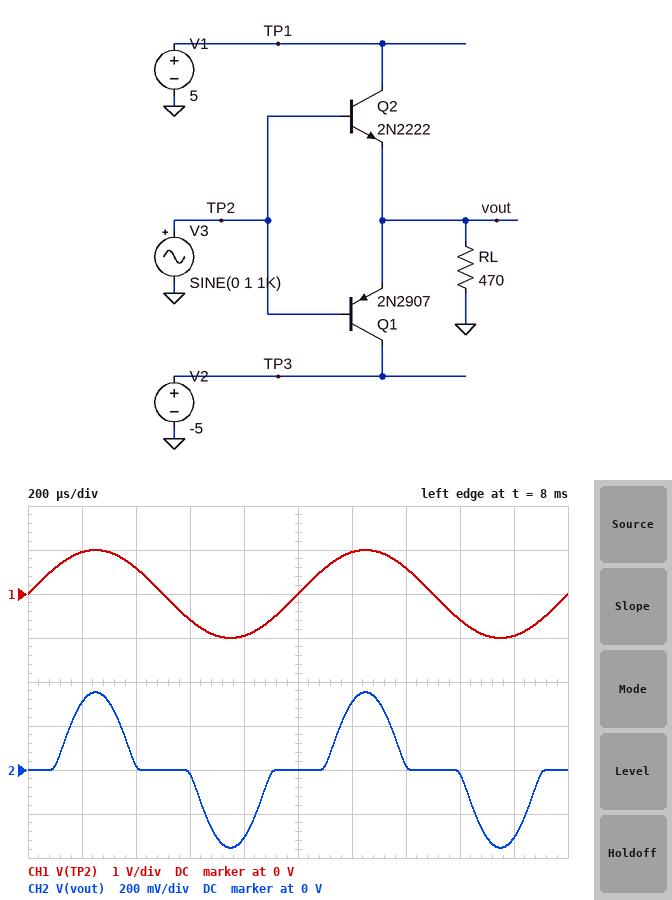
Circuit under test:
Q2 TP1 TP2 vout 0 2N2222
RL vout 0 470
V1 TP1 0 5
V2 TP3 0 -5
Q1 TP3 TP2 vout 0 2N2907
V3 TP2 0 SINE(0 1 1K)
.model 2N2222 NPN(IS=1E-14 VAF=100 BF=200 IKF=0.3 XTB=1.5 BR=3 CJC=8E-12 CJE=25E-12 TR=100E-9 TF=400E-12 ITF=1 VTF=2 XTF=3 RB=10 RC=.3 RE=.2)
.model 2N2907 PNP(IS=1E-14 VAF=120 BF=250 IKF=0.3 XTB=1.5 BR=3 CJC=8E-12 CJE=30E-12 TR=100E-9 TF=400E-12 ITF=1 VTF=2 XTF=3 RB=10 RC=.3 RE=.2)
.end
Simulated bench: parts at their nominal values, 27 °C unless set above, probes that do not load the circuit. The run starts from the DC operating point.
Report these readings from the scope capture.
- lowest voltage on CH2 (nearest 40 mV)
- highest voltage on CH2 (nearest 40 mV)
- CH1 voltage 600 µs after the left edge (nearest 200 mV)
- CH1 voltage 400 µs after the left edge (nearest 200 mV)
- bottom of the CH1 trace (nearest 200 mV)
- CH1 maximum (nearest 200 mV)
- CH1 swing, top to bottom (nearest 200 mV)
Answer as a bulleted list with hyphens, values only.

- -360 mV
- 360 mV
- -600 mV
- 600 mV
- -1.0 V
- 1.0 V
- 2.0 V
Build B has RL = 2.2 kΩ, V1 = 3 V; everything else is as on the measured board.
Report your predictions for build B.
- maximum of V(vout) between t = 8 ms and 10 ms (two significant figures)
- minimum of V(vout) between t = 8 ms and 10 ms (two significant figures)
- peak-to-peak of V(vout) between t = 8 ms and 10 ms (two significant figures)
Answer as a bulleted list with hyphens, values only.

- 390 mV
- -390 mV
- 780 mV
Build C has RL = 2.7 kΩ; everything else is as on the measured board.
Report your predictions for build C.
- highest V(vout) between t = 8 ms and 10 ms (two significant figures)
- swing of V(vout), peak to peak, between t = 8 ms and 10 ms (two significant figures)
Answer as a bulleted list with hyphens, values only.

- 400 mV
- 790 mV
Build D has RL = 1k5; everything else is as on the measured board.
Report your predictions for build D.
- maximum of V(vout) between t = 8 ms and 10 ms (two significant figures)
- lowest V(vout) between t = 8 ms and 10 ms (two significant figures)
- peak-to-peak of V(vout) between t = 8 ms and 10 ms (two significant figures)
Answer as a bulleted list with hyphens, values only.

- 380 mV
- -380 mV
- 760 mV
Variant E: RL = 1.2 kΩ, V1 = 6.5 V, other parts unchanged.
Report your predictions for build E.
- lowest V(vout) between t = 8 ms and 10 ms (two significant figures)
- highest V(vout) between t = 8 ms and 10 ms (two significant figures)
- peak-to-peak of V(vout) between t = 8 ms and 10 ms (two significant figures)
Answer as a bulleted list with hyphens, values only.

- -380 mV
- 380 mV
- 750 mV
